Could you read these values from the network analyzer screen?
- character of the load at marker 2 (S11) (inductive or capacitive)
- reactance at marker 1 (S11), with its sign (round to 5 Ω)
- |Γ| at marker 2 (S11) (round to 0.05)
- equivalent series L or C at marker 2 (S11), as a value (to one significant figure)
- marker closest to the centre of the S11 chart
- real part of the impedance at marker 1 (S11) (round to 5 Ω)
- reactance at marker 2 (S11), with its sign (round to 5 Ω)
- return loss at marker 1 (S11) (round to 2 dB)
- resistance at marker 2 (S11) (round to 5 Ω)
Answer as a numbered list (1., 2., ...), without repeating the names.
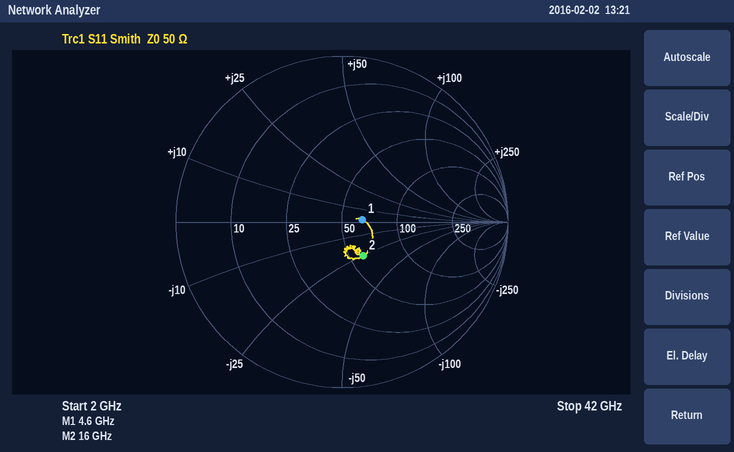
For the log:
1. capacitive
2. 0 Ω
3. 0.25
4. 400 fF
5. marker 1
6. 65 Ω
7. -25 Ω
8. 18 dB
9. 60 Ω
